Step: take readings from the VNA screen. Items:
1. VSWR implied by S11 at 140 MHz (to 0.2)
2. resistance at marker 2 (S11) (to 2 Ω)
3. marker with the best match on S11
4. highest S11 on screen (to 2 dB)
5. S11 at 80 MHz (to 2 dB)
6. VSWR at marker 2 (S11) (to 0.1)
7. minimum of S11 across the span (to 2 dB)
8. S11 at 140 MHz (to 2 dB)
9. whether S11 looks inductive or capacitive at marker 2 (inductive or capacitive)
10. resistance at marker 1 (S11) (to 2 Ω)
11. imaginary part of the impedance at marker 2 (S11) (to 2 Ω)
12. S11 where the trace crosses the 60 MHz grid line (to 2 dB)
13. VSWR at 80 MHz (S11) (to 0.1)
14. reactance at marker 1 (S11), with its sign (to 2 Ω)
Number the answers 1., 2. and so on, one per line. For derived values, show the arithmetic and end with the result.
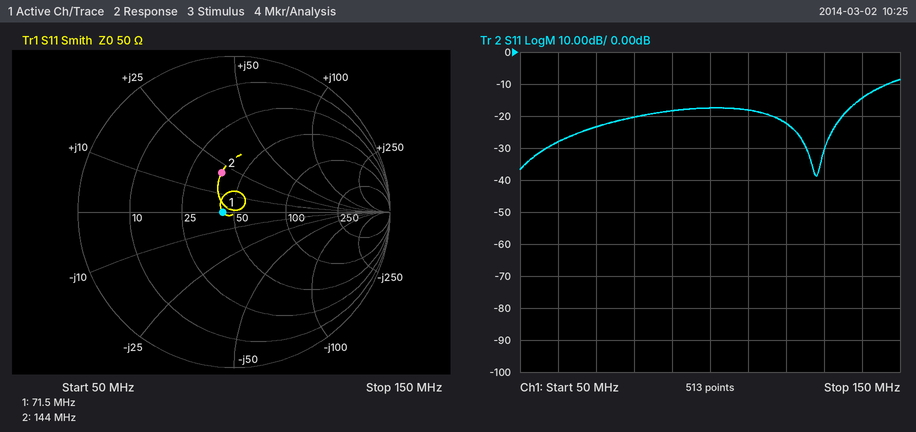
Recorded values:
1. |Γ| = 10^(-14/20) = 0.1995; VSWR = (1 + 0.1995)/(1 − 0.1995) ≈ 1.50, so 1.4 to the nearest 0.2
2. 38 Ω
3. marker 1
4. -8 dB
5. -20 dB
6. 1.7
7. -38 dB
8. -14 dB
9. inductive
10. 44 Ω
11. +20 Ω
12. -28 dB
13. |Γ| = 10^(-20/20) = 0.1000; VSWR = (1 + 0.1000)/(1 − 0.1000) ≈ 1.2
14. 0 Ω
